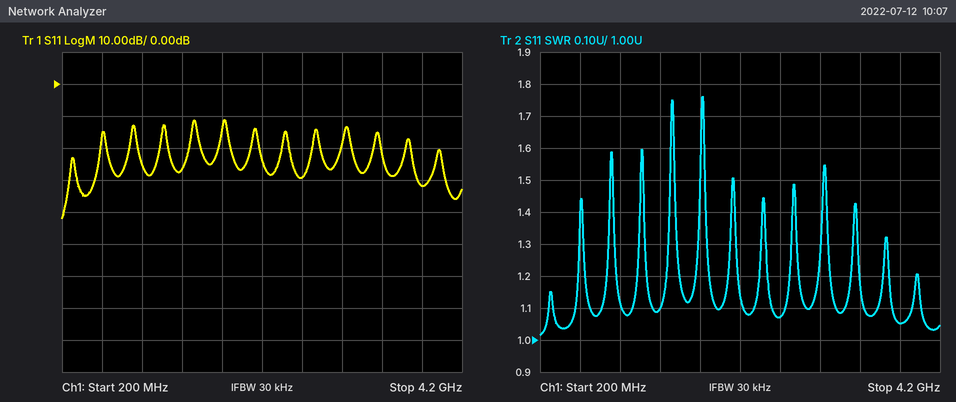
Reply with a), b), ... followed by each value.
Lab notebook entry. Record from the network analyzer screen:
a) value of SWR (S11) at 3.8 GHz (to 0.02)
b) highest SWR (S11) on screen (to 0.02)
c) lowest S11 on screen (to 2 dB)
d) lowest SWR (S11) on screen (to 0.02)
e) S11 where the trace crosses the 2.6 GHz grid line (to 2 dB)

a) 1.06
b) 1.76
c) -42 dB
d) 1.02
e) -30 dB
